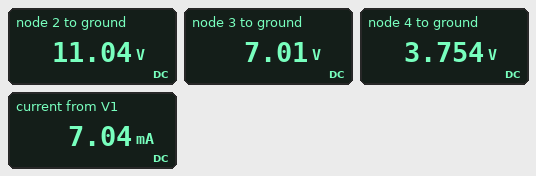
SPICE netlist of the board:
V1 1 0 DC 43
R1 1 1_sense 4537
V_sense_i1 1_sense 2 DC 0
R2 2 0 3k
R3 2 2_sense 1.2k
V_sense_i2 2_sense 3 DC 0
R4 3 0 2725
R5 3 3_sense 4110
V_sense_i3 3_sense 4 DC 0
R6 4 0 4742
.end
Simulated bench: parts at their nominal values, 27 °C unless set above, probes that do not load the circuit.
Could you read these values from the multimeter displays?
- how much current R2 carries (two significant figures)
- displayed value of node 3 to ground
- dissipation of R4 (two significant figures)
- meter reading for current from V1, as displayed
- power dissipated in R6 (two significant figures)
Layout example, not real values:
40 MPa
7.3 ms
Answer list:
3.7 mA
7.01 V
18 mW
7.04 mA
3.0 mW
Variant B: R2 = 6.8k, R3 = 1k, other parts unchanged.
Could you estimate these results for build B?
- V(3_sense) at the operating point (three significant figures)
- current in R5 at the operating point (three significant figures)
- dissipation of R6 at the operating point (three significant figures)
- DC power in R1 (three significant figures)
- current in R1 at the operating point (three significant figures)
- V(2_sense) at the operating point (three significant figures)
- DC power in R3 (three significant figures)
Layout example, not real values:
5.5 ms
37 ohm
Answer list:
4.96 V
1.05 mA
5.19 mW
189 mW
6.46 mA
9.26 V
19.7 mW
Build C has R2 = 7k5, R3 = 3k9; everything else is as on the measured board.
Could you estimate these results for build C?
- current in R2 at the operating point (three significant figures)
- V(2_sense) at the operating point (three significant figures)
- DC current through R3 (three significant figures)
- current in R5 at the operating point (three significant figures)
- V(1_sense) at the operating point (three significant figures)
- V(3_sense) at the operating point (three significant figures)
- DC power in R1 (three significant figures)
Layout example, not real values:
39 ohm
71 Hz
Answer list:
2.43 mA
6.34 V
3.04 mA
716 µA
18.2 V
3.39 V
136 mW
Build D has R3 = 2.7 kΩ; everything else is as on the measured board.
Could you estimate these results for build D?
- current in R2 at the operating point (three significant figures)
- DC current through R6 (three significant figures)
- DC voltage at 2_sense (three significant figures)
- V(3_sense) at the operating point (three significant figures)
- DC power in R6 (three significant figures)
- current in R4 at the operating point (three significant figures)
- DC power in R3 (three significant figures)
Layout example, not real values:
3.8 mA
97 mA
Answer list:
4.14 mA
611 µA
5.41 V
2.90 V
1.77 mW
1.99 mA
18.2 mW
